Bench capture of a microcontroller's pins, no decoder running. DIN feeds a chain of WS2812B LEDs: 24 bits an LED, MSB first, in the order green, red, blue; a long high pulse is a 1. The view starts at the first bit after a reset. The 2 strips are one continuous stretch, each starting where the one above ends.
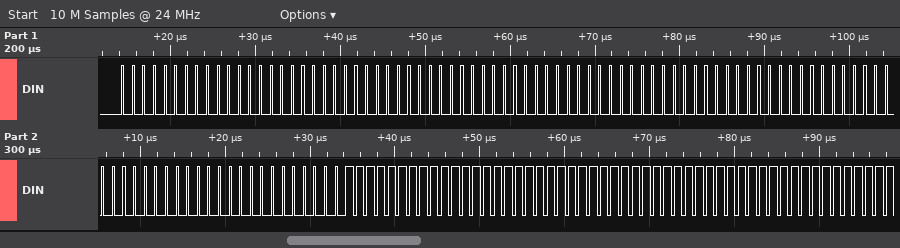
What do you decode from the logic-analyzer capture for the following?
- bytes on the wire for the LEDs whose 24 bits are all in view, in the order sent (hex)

00 00 00 00 00 00 00 00 00 00 00 00 FF FF FF FF FF FF
